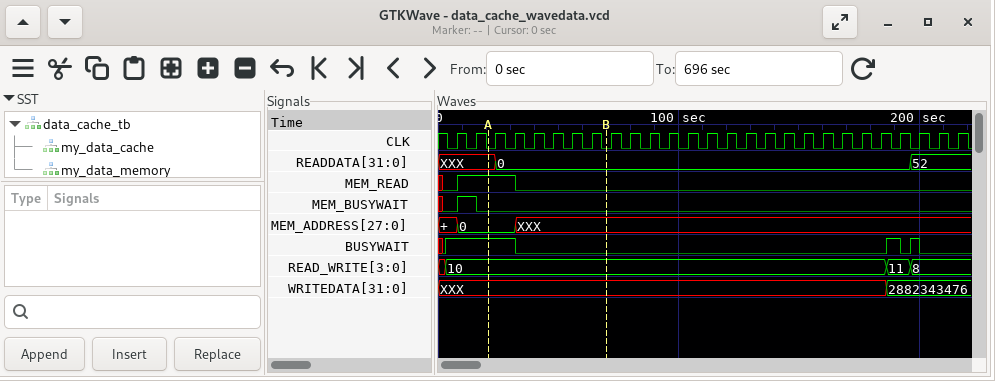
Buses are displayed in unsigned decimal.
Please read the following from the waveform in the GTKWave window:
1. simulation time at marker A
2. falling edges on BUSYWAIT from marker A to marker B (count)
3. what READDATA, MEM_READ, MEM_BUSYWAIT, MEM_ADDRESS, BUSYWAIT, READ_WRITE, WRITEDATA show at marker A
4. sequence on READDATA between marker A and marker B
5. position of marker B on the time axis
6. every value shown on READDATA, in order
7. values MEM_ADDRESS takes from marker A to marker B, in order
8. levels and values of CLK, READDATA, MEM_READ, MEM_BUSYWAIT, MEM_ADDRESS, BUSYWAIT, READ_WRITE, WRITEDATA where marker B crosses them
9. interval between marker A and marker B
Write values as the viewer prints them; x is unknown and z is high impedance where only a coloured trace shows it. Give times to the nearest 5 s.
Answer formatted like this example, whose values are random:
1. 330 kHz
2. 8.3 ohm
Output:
1. 20 s
2. 1
3. READDATA=XXX, MEM_READ=1, MEM_BUSYWAIT=0, MEM_ADDRESS=0, BUSYWAIT=1, READ_WRITE=10, WRITEDATA=XXX
4. XXX, 0
5. 70 s
6. XXX, 0, 52
7. 0, XXX
8. CLK=0, READDATA=0, MEM_READ=0, MEM_BUSYWAIT=0, MEM_ADDRESS=XXX, BUSYWAIT=0, READ_WRITE=10, WRITEDATA=XXX
9. 50 s
